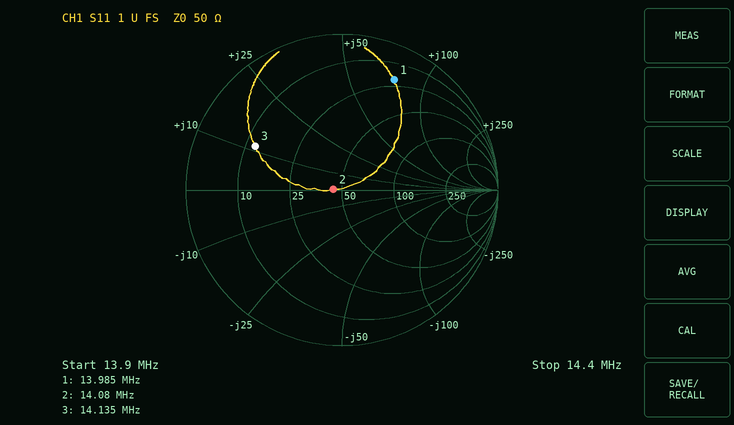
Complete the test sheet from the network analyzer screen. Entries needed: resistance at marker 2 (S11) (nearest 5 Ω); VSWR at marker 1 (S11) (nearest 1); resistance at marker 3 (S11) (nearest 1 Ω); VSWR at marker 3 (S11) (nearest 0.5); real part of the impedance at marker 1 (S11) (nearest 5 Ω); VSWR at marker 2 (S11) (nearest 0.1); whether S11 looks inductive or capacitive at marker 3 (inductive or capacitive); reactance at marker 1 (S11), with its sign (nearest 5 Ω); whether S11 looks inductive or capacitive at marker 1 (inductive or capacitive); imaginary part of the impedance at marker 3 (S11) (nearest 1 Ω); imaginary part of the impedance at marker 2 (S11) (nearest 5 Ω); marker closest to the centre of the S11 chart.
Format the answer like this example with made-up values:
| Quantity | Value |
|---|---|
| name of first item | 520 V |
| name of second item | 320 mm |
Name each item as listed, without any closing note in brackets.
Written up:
| Quantity | Value |
|---|---|
| resistance at marker 2 (S11) | 45 Ω |
| VSWR at marker 1 (S11) | 8 |
| resistance at marker 3 (S11) | 12 Ω |
| VSWR at marker 3 (S11) | 4.5 |
| real part of the impedance at marker 1 (S11) | 20 Ω |
| VSWR at marker 2 (S11) | 1.1 |
| whether S11 looks inductive or capacitive at marker 3 | inductive |
| reactance at marker 1 (S11), with its sign | +75 Ω |
| whether S11 looks inductive or capacitive at marker 1 | inductive |
| imaginary part of the impedance at marker 3 (S11) | +11 Ω |
| imaginary part of the impedance at marker 2 (S11) | 0 Ω |
| marker closest to the centre of the S11 chart | marker 2 |
